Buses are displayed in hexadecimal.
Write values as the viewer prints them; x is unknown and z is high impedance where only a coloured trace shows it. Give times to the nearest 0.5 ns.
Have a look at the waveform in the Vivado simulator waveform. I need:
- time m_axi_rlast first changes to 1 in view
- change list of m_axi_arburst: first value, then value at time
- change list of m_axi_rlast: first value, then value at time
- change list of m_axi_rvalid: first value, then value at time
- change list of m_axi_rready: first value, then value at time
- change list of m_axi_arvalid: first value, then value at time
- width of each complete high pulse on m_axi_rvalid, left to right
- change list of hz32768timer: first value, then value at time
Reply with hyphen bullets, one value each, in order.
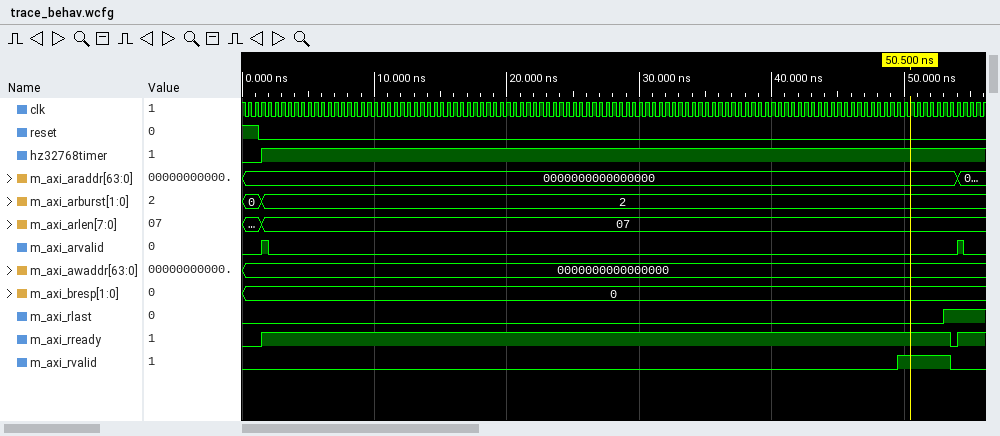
- 53 ns
- 0, 2 at 1.5 ns
- 0, 1 at 53 ns
- 0, 1 at 49.5 ns, 0 at 53.5 ns
- 0, 1 at 1.5 ns, 0 at 53.5 ns, 1 at 54 ns
- 0, 1 at 1.5 ns, 0 at 2 ns, 1 at 54 ns, 0 at 54.5 ns
- 4 ns
- 0, 1 at 1.5 ns
